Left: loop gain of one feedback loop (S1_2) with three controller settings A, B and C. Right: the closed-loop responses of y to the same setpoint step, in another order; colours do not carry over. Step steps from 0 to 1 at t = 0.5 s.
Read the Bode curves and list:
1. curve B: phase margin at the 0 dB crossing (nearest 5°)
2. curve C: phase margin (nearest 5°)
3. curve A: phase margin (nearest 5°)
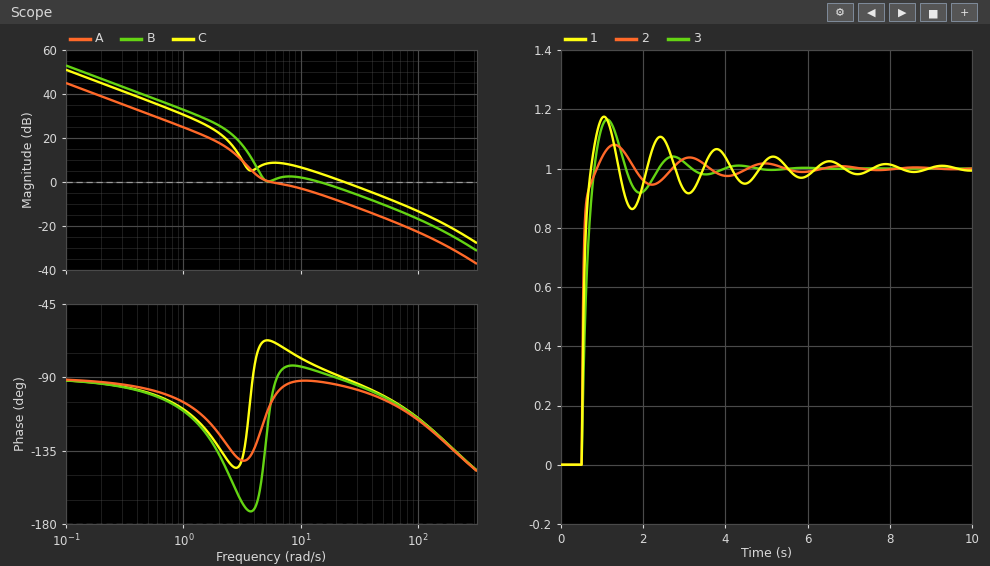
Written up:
95°
90°
75°
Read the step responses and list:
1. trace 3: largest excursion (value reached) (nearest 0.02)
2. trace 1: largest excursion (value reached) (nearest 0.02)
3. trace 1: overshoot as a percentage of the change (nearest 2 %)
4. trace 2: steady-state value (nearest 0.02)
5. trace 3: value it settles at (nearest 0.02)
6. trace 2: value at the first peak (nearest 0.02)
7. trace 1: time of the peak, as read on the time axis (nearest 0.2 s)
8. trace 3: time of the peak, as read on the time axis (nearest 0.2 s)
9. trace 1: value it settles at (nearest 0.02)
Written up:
1.16
1.18
18 %
1.00
1.00
1.08
1.0 s
1.2 s
1.00
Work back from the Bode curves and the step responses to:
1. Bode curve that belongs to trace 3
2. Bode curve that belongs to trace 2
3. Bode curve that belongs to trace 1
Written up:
A
C
B
